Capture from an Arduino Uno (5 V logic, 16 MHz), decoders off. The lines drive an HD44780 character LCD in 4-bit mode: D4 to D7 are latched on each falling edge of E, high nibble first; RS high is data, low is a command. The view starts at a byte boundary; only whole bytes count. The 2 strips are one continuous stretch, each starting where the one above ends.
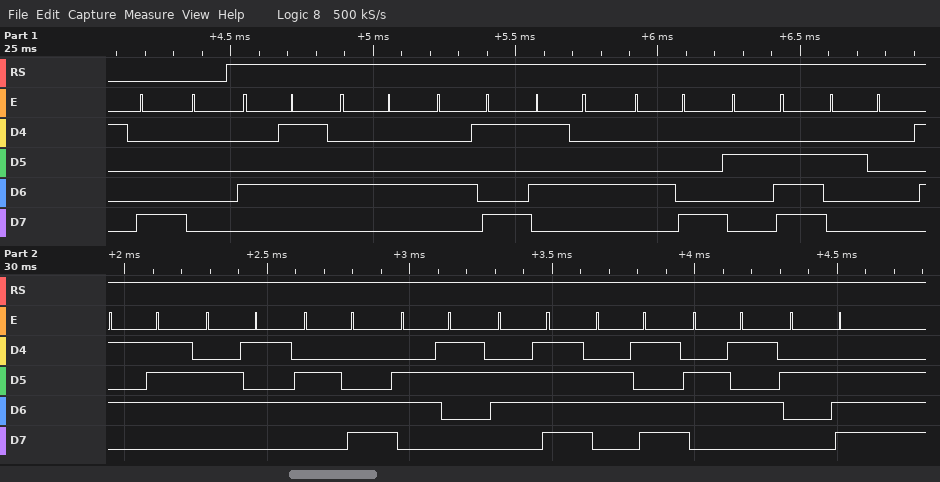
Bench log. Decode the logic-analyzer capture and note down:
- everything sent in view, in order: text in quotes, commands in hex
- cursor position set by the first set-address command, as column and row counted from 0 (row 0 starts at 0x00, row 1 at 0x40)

0x80 "EDITH. Welcome."
column 0, row 0
